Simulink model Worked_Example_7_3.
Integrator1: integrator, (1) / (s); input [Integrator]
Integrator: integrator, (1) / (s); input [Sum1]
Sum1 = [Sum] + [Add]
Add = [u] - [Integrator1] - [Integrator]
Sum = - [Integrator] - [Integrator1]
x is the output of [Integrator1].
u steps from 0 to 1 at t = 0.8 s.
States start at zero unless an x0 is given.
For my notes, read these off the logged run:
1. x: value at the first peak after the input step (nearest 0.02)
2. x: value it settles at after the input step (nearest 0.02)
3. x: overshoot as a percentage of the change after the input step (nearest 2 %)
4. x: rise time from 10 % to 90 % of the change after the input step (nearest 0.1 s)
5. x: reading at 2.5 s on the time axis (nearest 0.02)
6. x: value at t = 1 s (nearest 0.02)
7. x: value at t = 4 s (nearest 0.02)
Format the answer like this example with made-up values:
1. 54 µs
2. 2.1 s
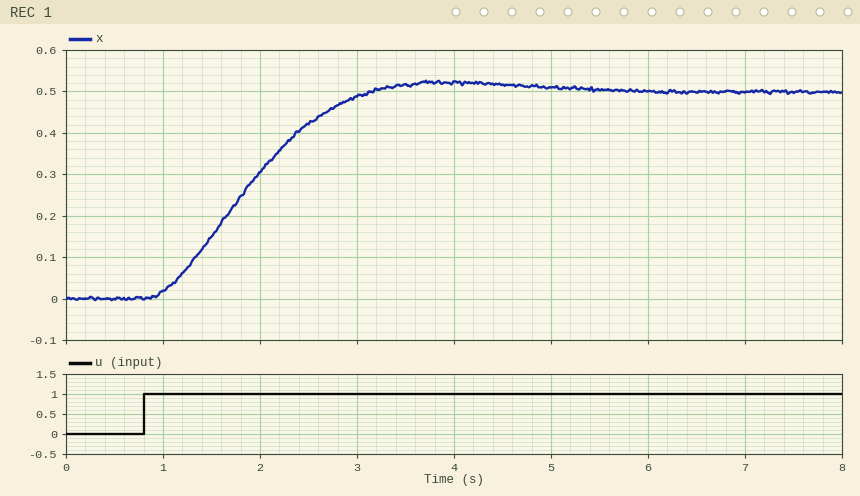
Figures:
1. 0.52
2. 0.50
3. 4 %
4. 1.5 s
5. 0.42
6. 0.02
7. 0.52
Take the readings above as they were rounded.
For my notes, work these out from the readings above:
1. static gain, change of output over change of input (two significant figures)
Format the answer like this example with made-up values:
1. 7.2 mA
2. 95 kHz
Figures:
1. 0.50
